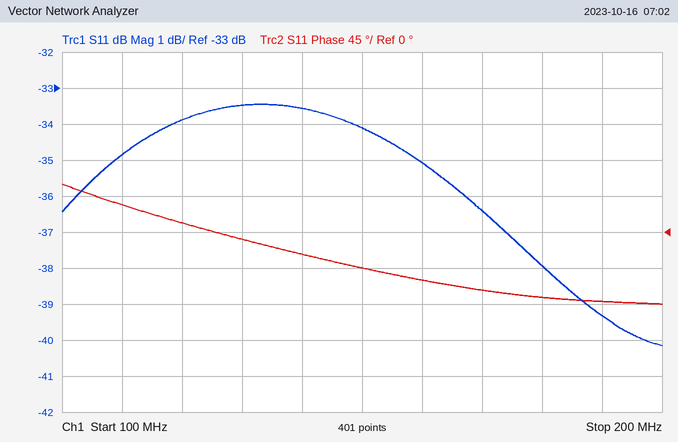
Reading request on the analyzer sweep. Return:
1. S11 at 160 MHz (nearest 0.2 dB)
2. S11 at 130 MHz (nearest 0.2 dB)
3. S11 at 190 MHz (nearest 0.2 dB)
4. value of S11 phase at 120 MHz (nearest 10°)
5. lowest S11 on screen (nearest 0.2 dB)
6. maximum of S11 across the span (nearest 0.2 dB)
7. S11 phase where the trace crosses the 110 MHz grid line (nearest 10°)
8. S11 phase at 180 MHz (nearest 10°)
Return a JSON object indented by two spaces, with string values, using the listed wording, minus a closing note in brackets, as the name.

{
  "S11 at 160 MHz": "-35.0 dB",
  "S11 at 130 MHz": "-33.4 dB",
  "S11 at 190 MHz": "-39.4 dB",
  "value of S11 phase at 120 MHz": "10°",
  "lowest S11 on screen": "-40.2 dB",
  "maximum of S11 across the span": "-33.4 dB",
  "S11 phase where the trace crosses the 110 MHz grid line": "30°",
  "S11 phase at 180 MHz": "-80°"
}
